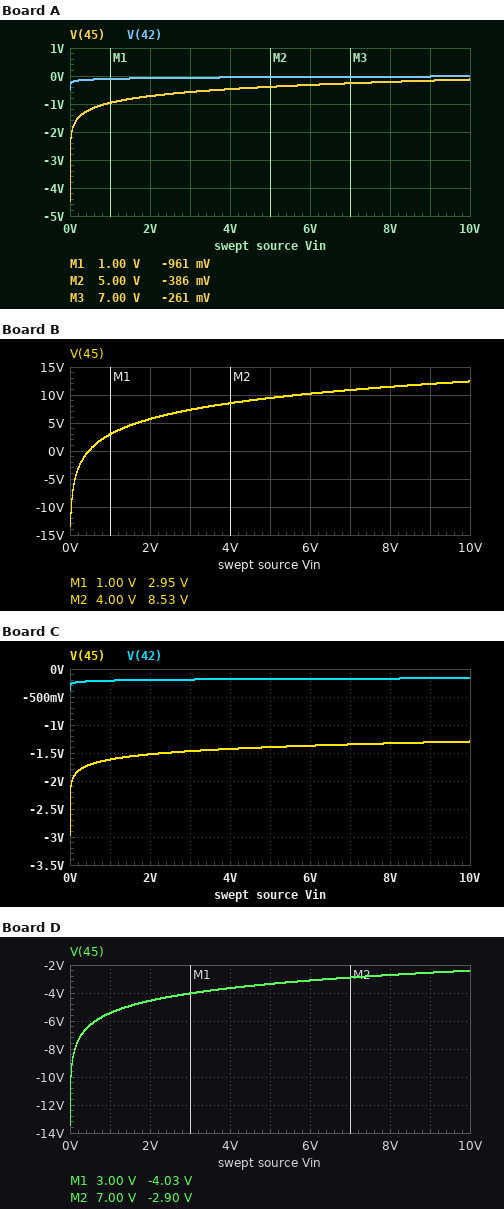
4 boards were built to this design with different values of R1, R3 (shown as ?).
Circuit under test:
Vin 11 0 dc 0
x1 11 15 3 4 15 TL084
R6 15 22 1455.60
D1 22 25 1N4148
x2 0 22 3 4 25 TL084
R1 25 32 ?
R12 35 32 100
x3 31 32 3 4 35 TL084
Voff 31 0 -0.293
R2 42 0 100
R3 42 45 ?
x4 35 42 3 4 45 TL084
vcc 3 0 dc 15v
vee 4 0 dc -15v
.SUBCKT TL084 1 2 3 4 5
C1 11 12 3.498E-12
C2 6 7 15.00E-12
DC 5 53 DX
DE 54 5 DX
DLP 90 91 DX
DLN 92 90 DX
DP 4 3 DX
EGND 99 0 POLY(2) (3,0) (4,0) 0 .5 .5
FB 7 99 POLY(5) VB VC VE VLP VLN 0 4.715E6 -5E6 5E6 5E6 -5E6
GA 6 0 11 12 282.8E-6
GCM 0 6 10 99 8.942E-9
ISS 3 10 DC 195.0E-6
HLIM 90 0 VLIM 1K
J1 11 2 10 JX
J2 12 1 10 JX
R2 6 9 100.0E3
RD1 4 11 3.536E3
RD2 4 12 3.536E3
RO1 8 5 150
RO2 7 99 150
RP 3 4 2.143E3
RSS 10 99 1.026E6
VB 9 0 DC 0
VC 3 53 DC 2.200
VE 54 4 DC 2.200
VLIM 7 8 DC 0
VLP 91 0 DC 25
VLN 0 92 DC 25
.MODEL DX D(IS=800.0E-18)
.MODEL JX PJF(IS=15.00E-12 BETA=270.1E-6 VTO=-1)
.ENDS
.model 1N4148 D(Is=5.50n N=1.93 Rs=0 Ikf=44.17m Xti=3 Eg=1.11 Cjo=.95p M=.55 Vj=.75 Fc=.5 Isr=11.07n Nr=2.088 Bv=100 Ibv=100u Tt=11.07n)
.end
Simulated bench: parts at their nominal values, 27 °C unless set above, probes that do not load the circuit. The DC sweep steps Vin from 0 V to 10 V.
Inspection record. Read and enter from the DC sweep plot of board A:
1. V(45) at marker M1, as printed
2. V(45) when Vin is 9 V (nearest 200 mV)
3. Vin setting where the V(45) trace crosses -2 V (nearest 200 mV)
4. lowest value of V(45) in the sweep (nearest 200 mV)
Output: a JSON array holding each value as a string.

["-961 mV", "-200 mV", "0 V", "-4.4 V"]
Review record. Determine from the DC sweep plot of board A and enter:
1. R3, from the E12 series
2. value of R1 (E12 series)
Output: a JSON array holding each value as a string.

["820 Ω", "150 Ω"]
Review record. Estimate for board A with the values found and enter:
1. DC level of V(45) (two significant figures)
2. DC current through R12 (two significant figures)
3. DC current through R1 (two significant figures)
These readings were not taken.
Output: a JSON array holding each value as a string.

["-4.5 V", "1.9 mA", "1.9 mA"]
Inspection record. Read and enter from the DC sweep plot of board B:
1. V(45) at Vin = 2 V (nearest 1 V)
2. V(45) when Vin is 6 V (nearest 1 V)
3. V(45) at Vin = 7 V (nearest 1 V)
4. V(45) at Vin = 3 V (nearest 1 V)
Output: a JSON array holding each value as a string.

["6 V", "10 V", "11 V", "7 V"]
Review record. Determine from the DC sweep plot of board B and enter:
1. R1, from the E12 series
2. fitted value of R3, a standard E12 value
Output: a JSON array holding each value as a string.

["82 Ω", "5.6 kΩ"]
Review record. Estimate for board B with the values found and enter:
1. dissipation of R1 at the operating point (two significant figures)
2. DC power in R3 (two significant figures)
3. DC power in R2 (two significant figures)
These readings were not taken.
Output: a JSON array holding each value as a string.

["980 µW", "31 mW", "560 µW"]
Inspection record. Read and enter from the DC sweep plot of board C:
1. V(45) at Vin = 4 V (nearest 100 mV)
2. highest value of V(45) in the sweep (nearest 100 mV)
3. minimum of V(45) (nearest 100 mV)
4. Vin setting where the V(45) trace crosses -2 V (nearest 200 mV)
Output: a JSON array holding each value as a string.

["-1.4 V", "-1.3 V", "-3.0 V", "0 V"]
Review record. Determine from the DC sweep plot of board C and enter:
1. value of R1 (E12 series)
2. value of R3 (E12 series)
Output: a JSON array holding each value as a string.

["330 Ω", "680 Ω"]
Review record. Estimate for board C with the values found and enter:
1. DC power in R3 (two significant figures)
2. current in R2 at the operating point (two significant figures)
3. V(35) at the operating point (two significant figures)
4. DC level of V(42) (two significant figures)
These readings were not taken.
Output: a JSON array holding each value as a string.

["9.9 mW", "3.8 mA", "-380 mV", "-380 mV"]
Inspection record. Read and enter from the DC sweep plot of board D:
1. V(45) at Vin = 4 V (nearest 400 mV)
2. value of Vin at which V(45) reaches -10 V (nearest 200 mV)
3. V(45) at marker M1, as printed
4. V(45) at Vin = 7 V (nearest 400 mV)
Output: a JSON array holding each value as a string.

["-3.6 V", "0 V", "-4.03 V", "-2.8 V"]
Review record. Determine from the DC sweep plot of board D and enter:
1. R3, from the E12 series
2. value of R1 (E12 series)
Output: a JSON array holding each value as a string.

["3.9 kΩ", "180 Ω"]
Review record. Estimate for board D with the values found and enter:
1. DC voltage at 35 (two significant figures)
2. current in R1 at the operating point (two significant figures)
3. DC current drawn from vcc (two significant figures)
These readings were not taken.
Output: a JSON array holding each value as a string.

["-450 mV", "1.6 mA", "57 mA"]
